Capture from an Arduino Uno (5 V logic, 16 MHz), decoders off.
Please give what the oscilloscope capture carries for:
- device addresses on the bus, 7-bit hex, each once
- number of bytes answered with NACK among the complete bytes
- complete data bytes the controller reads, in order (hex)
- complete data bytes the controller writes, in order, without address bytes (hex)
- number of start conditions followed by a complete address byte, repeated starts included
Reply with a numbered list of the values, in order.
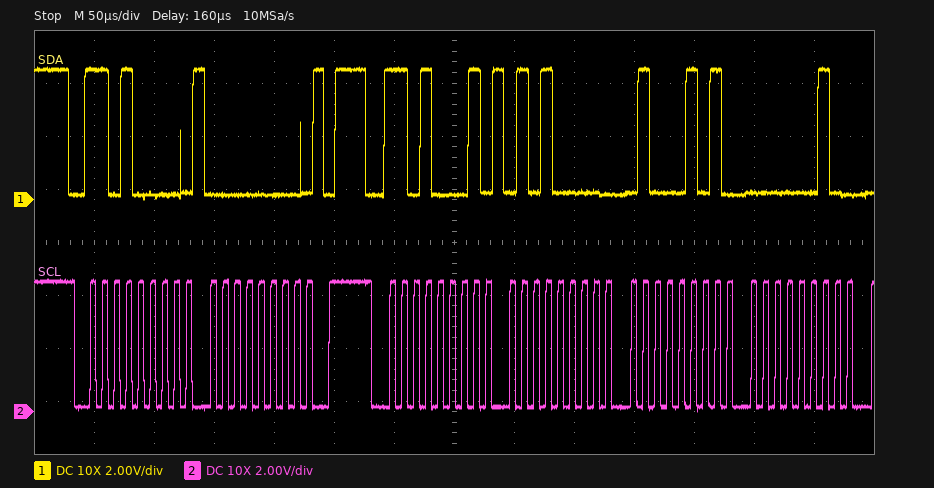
1. 0x68
2. 0
3. 50 45 02
4. 00
5. 2
